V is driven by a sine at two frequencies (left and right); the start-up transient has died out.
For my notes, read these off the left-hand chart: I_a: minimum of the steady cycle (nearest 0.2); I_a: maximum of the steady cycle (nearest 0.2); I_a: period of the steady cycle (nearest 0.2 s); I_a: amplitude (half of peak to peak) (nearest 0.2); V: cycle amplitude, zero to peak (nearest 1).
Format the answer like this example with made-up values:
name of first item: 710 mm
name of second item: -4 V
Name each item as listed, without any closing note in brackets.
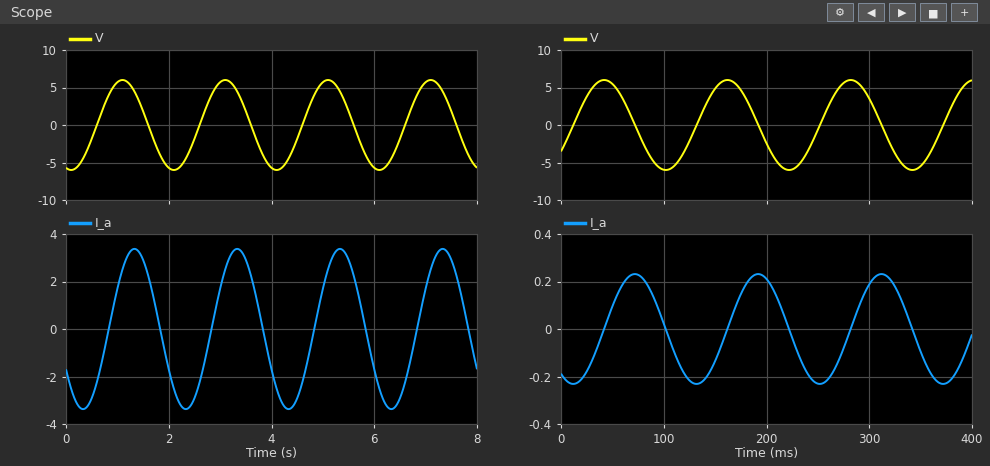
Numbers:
I_a: minimum of the steady cycle: -3.4
I_a: maximum of the steady cycle: 3.4
I_a: period of the steady cycle: 2.0 s
I_a: amplitude (half of peak to peak): 3.4
V: cycle amplitude, zero to peak: 6
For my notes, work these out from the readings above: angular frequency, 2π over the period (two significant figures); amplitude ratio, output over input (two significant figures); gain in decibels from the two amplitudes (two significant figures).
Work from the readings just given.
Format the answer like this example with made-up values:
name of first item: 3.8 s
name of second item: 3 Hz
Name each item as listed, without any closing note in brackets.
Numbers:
angular frequency, 2π over the period: 3.1 rad/s
amplitude ratio, output over input: 0.57
gain in decibels from the two amplitudes: -4.9 dB
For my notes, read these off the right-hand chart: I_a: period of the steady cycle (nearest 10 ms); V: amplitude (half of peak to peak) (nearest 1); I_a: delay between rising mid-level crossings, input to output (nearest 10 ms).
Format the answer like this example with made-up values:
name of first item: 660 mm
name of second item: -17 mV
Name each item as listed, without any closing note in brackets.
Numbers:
I_a: period of the steady cycle: 120 ms
V: amplitude (half of peak to peak): 6
I_a: delay between rising mid-level crossings, input to output: 30 ms
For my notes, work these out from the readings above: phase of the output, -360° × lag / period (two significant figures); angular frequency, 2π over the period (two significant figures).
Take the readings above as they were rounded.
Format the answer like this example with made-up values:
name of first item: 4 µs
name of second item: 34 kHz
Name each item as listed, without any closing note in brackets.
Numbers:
phase of the output, -360° × lag / period: -90°
angular frequency, 2π over the period: 0.052 rad/ms
